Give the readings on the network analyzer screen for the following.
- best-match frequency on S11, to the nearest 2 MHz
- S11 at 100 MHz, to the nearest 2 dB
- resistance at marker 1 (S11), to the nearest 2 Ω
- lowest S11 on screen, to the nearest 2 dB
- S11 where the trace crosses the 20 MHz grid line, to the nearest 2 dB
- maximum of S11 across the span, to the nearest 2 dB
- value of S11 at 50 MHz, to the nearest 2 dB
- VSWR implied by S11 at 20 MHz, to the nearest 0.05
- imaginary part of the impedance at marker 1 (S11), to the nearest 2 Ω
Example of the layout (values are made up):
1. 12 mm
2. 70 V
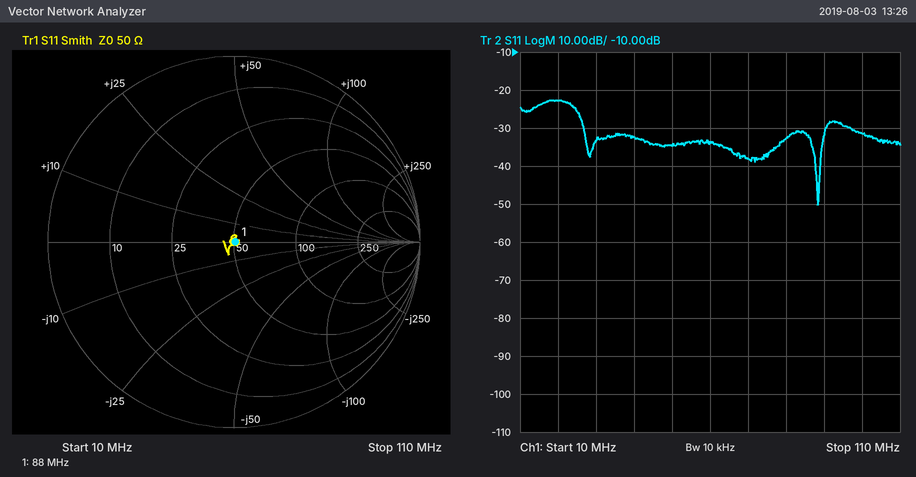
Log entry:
1. 88 MHz
2. -32 dB
3. 50 Ω
4. -50 dB
5. -22 dB
6. -22 dB
7. -34 dB
8. 1.15
9. 0 Ω
